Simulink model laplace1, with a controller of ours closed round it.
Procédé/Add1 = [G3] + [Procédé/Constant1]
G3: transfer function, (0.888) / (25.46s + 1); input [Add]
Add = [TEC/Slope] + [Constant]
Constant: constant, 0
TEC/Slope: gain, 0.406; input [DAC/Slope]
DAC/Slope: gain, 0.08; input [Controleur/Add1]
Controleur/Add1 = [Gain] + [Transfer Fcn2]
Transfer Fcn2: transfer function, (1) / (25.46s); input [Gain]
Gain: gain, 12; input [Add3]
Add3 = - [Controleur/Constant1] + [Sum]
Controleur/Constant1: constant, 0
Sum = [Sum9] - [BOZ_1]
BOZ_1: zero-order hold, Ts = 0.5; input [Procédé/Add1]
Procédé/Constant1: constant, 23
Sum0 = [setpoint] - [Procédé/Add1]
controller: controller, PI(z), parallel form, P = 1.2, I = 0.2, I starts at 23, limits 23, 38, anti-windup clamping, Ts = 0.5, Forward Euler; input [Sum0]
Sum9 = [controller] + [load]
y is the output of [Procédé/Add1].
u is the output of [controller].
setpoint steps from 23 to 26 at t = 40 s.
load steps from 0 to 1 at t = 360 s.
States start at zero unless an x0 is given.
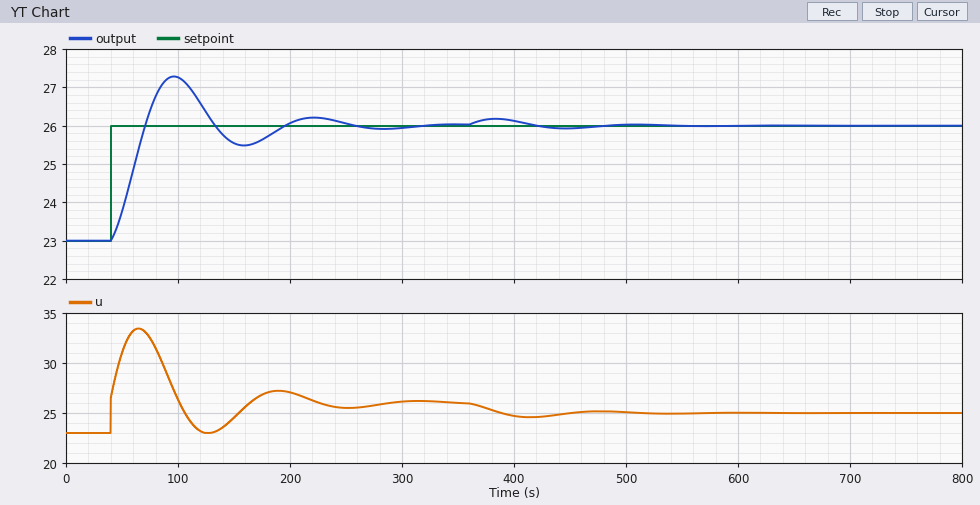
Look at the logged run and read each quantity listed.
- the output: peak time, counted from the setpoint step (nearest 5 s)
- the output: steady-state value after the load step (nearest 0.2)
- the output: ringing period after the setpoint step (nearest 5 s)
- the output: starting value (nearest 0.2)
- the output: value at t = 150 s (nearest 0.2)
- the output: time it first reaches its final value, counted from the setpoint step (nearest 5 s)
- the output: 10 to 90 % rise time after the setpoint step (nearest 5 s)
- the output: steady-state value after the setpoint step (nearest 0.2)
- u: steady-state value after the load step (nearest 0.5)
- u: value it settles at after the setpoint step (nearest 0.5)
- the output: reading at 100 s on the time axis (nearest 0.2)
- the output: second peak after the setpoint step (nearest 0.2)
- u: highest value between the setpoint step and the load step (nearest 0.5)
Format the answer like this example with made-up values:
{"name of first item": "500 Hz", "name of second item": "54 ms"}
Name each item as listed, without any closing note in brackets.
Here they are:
{"the output: peak time, counted from the setpoint step": "55 s", "the output: steady-state value after the load step": "26.0", "the output: ringing period after the setpoint step": "125 s", "the output: starting value": "23.0", "the output: value at t = 150 s": "25.6", "the output: time it first reaches its final value, counted from the setpoint step": "30 s", "the output: 10 to 90 % rise time after the setpoint step": "25 s", "the output: steady-state value after the setpoint step": "26.0", "u: steady-state value after the load step": "25.0", "u: value it settles at after the setpoint step": "26.0", "the output: reading at 100 s on the time axis": "27.2", "the output: second peak after the setpoint step": "26.2", "u: highest value between the setpoint step and the load step": "33.5"}
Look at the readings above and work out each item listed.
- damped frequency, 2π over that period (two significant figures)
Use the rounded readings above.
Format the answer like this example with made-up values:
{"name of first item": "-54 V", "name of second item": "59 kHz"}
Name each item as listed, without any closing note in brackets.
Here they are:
{"damped frequency, 2π over that period": "0.050 rad/s"}
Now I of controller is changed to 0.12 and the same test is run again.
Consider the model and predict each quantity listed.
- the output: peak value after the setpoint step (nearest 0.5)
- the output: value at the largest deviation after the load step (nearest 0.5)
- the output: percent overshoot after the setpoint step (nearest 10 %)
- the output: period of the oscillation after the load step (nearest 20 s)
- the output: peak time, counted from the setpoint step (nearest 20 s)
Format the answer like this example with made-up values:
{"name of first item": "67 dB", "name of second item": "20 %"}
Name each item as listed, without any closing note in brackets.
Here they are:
{"the output: peak value after the setpoint step": "27.0", "the output: value at the largest deviation after the load step": "26.0", "the output: percent overshoot after the setpoint step": "30 %", "the output: period of the oscillation after the load step": "160 s", "the output: peak time, counted from the setpoint step": "80 s"}
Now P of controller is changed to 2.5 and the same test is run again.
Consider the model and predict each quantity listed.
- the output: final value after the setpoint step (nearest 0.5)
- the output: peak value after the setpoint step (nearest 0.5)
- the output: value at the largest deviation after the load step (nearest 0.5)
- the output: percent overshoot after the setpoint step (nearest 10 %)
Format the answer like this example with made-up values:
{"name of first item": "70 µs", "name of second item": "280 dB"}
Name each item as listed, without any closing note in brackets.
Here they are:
{"the output: final value after the setpoint step": "26.0", "the output: peak value after the setpoint step": "27.0", "the output: value at the largest deviation after the load step": "26.0", "the output: percent overshoot after the setpoint step": "30 %"}
